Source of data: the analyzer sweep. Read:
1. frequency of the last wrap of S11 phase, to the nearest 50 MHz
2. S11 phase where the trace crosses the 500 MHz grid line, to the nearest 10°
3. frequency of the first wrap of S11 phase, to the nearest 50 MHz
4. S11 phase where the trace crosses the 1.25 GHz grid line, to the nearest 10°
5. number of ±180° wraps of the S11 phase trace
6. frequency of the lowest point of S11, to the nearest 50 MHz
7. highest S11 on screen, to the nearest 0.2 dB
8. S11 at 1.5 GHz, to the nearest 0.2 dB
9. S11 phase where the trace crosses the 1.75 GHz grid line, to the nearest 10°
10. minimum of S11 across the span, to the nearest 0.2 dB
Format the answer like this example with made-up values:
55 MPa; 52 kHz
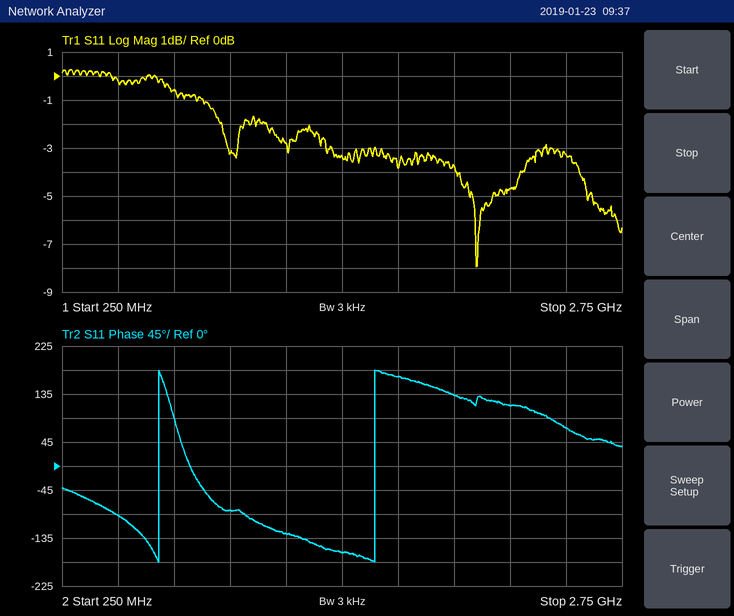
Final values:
1.65 GHz; -90°; 700 MHz; -130°; 2; 2.10 GHz; 0.2 dB; -3.4 dB; 170°; -8.0 dB
